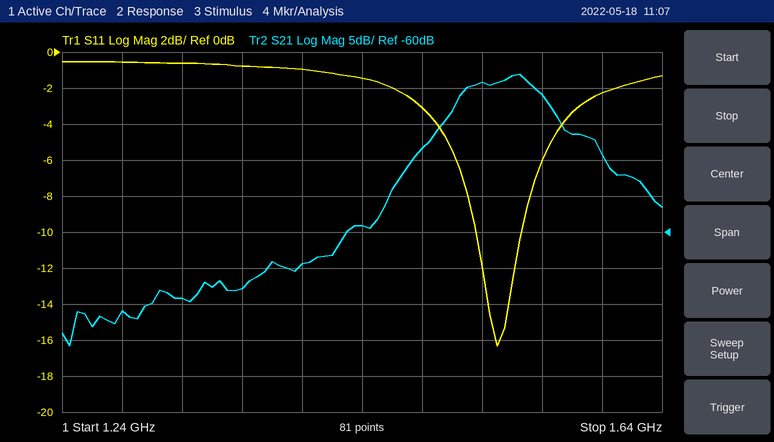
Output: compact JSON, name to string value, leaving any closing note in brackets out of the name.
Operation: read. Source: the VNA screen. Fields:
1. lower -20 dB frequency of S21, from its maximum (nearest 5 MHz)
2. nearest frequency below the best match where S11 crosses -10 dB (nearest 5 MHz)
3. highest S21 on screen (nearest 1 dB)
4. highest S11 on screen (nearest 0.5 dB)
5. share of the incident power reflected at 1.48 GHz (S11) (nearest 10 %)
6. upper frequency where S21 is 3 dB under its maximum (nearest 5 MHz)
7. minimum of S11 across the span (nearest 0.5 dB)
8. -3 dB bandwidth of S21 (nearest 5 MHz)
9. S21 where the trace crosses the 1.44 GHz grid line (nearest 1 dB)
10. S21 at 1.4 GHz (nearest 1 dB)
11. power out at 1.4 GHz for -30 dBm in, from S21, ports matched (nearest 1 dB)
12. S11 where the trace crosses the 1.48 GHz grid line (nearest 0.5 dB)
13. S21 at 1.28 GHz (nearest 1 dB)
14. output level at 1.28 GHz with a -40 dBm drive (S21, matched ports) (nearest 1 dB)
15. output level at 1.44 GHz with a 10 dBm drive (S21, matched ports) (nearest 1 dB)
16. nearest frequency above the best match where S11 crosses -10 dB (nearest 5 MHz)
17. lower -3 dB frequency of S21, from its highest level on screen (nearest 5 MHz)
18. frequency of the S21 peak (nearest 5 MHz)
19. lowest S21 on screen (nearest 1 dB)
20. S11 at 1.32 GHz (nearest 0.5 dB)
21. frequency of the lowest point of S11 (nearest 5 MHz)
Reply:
{"lower -20 dB frequency of S21, from its maximum": "1.450 GHz", "nearest frequency below the best match where S11 crosses -10 dB": "1.515 GHz", "highest S21 on screen": "-38 dB", "highest S11 on screen": "-0.5 dB", "share of the incident power reflected at 1.48 GHz (S11)": "50 %", "upper frequency where S21 is 3 dB under its maximum": "1.560 GHz", "minimum of S11 across the span": "-16.5 dB", "-3 dB bandwidth of S21": "55 MHz", "S21 where the trace crosses the 1.44 GHz grid line": "-59 dB", "S21 at 1.4 GHz": "-64 dB", "power out at 1.4 GHz for -30 dBm in, from S21, ports matched": "-94 dBm", "S11 where the trace crosses the 1.48 GHz grid line": "-3.0 dB", "S21 at 1.28 GHz": "-71 dB", "output level at 1.28 GHz with a -40 dBm drive (S21, matched ports)": "-111 dBm", "output level at 1.44 GHz with a 10 dBm drive (S21, matched ports)": "-49 dBm", "nearest frequency above the best match where S11 crosses -10 dB": "1.545 GHz", "lower -3 dB frequency of S21, from its highest level on screen": "1.505 GHz", "frequency of the S21 peak": "1.545 GHz", "lowest S21 on screen": "-76 dB", "S11 at 1.32 GHz": "-0.5 dB", "frequency of the lowest point of S11": "1.530 GHz"}
